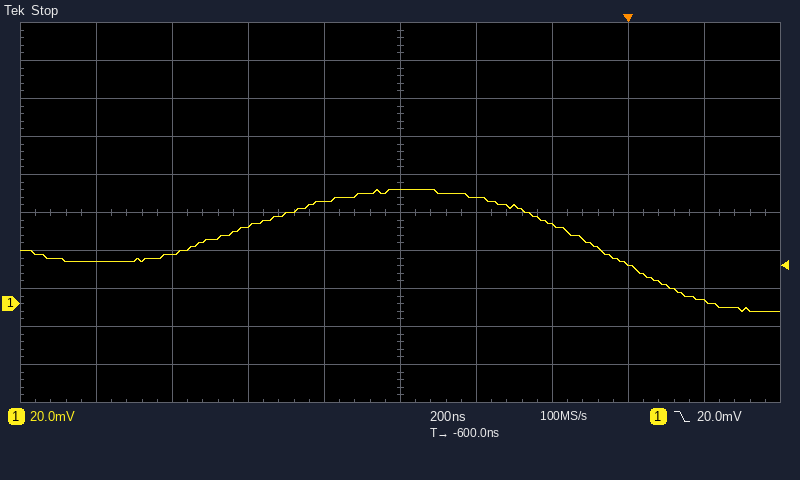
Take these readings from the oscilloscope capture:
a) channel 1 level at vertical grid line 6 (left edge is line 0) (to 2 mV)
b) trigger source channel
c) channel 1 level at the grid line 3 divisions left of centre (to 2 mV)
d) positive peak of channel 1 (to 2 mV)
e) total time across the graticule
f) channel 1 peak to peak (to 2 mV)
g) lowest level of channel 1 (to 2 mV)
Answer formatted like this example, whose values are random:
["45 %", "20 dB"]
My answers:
["56 mV", "channel 1", "26 mV", "60 mV", "2 µs", "64 mV", "-4 mV"]
